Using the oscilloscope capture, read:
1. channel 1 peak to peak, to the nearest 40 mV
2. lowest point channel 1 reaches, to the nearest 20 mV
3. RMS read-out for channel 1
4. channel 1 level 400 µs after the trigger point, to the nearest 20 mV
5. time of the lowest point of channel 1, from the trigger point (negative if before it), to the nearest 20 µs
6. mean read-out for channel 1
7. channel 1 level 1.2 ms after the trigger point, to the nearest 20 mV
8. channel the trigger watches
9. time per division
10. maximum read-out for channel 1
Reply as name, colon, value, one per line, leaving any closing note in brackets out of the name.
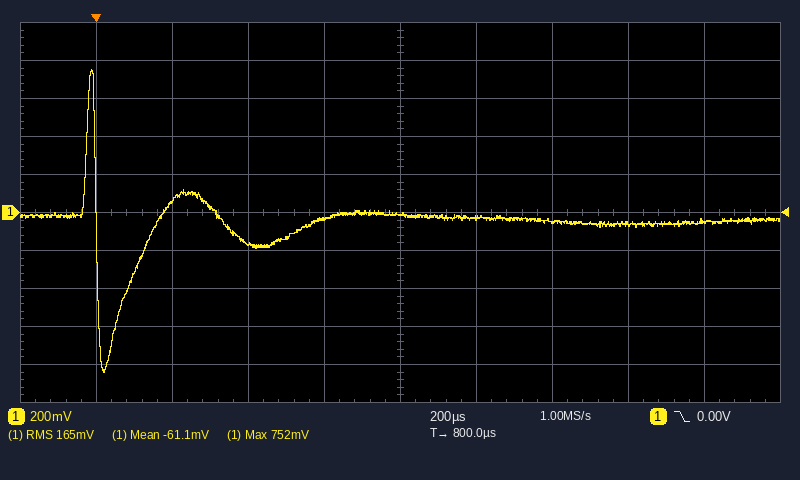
channel 1 peak to peak, to the nearest 40 mV: 1.60 V
lowest point channel 1 reaches, to the nearest 20 mV: -840 mV
RMS read-out for channel 1: 165 mV
channel 1 level 400 µs after the trigger point, to the nearest 20 mV: -160 mV
time of the lowest point of channel 1, from the trigger point (negative if before it), to the nearest 20 µs: +20 µs
mean read-out for channel 1: -61.1 mV
channel 1 level 1.2 ms after the trigger point, to the nearest 20 mV: -40 mV
channel the trigger watches: channel 1
time per division: 200 µs
maximum read-out for channel 1: 752 mV
